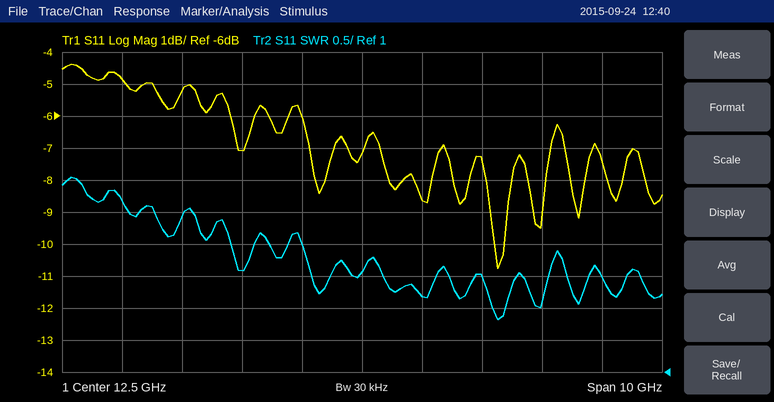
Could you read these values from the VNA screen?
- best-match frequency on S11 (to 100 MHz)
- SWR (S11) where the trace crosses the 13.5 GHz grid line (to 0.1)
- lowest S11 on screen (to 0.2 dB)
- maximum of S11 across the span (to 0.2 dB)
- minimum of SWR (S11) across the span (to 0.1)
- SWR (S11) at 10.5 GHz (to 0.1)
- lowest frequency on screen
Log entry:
14.8 GHz
2.2
-10.8 dB
-4.4 dB
1.8
2.6
7.5 GHz
